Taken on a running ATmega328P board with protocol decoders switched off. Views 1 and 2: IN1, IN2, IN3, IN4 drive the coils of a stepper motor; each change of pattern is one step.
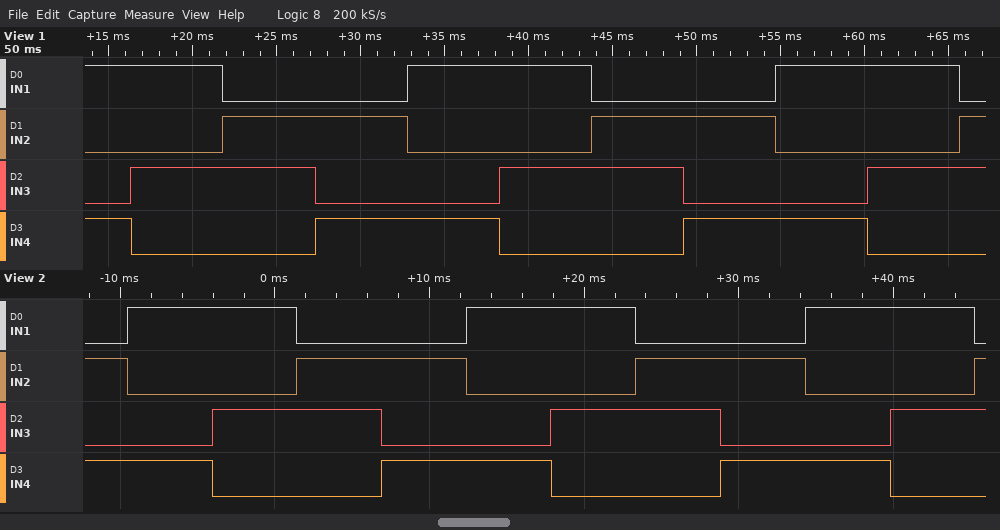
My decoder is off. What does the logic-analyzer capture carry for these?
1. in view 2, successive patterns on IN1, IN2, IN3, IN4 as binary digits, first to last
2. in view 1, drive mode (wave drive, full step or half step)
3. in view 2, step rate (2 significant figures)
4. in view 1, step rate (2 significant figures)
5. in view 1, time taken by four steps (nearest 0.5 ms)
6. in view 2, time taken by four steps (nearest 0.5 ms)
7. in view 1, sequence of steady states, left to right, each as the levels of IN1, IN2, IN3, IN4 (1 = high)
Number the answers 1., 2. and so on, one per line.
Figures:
1. 0101 1001 1010 0110 0101 1001 1010 0110 0101 1001 1010 0110
2. full step
3. 180 steps/s
4. 180 steps/s
5. 22.0 ms
6. 22.0 ms
7. 1001 1010 0110 0101 1001 1010 0110 0101 1001 1010 0110
